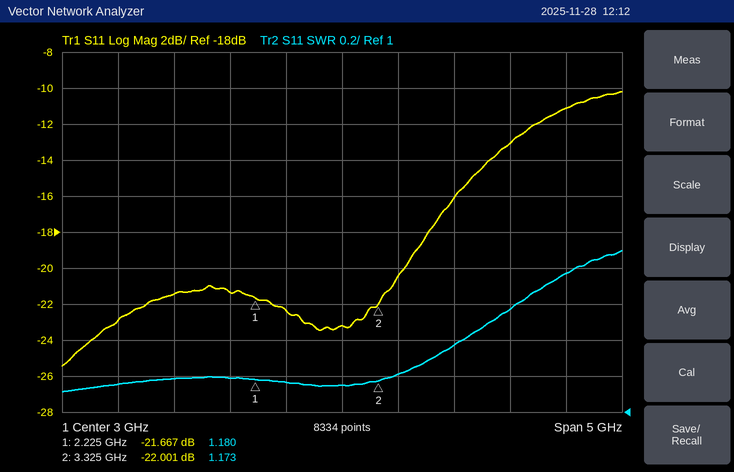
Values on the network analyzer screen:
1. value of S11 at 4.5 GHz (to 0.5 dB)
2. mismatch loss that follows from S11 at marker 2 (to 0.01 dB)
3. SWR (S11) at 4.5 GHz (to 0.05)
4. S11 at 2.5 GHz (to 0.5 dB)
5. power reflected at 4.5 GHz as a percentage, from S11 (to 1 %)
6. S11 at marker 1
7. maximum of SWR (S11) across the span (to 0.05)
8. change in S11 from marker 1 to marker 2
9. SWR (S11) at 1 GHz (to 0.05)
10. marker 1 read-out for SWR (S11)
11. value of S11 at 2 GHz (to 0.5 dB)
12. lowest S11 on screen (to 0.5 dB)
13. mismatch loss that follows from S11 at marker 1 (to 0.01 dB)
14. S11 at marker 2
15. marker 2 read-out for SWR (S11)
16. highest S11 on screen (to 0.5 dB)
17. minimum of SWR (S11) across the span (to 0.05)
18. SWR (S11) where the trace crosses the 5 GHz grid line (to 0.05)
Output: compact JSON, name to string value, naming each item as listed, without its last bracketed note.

{"value of S11 at 4.5 GHz": "-13.0 dB", "mismatch loss that follows from S11 at marker 2": "0.03 dB", "SWR (S11) at 4.5 GHz": "1.55", "S11 at 2.5 GHz": "-22.5 dB", "power reflected at 4.5 GHz as a percentage, from S11": "5 %", "S11 at marker 1": "-21.667 dB", "maximum of SWR (S11) across the span": "1.90", "change in S11 from marker 1 to marker 2": "-0.334 dB", "SWR (S11) at 1 GHz": "1.15", "marker 1 read-out for SWR": "1.180", "value of S11 at 2 GHz": "-21.5 dB", "lowest S11 on screen": "-25.5 dB", "mismatch loss that follows from S11 at marker 1": "0.03 dB", "S11 at marker 2": "-22.001 dB", "marker 2 read-out for SWR": "1.173", "highest S11 on screen": "-10.0 dB", "minimum of SWR (S11) across the span": "1.10", "SWR (S11) where the trace crosses the 5 GHz grid line": "1.75"}
